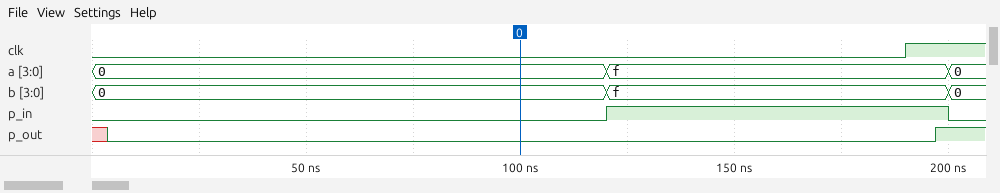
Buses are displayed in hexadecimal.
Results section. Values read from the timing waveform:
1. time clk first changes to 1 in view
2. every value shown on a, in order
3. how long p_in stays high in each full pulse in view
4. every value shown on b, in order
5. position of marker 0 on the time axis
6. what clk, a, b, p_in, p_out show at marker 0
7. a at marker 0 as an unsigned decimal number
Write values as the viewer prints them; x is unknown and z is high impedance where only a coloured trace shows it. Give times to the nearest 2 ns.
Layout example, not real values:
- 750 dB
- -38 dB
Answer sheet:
- 190 ns
- 0, f, 0
- 80 ns
- 0, f, 0
- 100 ns
- clk=0, a=0, b=0, p_in=0, p_out=0
- 0
